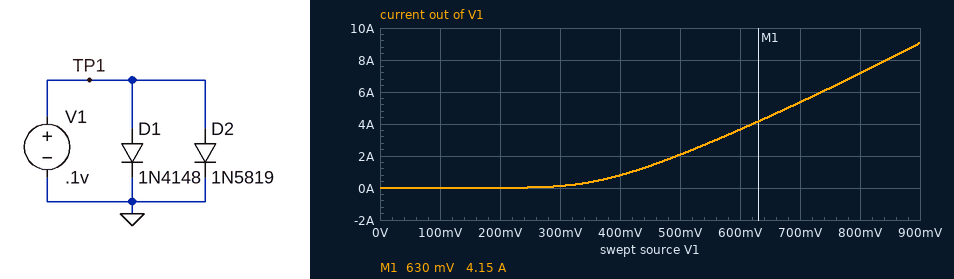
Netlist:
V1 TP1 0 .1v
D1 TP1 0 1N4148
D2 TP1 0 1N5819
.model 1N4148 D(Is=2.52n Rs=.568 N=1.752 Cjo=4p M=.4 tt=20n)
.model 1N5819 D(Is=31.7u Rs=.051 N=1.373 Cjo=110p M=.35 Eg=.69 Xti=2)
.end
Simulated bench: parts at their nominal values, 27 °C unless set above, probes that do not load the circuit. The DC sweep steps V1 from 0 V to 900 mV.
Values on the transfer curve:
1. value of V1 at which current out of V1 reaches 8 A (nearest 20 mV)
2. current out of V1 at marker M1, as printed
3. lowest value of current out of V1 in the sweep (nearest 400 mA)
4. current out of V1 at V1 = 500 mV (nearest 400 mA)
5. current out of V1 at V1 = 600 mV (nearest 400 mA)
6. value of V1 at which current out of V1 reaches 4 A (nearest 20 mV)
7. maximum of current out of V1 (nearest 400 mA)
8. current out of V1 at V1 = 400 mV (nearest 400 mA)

840 mV
4.15 A
0 A
2.0 A
3.6 A
620 mV
9.2 A
800 mA
